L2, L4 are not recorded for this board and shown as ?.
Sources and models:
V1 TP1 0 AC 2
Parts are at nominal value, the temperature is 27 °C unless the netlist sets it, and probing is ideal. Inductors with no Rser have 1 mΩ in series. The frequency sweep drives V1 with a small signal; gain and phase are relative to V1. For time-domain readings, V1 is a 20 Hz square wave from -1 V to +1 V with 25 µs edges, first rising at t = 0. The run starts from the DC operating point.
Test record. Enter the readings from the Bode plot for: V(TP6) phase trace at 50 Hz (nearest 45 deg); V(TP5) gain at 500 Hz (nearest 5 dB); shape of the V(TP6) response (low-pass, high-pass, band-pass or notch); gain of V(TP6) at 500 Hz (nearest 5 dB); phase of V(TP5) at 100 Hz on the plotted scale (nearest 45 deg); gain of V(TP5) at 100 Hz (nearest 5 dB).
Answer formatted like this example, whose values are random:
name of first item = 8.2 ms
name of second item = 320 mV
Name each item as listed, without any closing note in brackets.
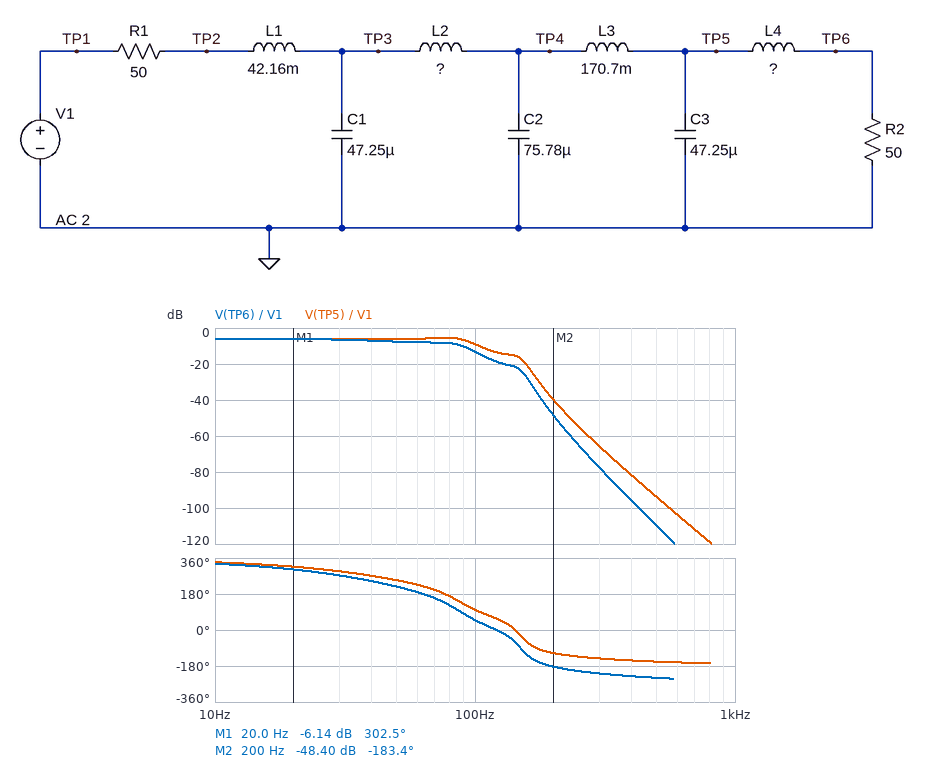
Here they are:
V(TP6) phase trace at 50 Hz = 225 deg
V(TP5) gain at 500 Hz = -95 dB
shape of the V(TP6) response = low-pass
gain of V(TP6) at 500 Hz = -110 dB
phase of V(TP5) at 100 Hz on the plotted scale = 90 deg
gain of V(TP5) at 100 Hz = -10 dB
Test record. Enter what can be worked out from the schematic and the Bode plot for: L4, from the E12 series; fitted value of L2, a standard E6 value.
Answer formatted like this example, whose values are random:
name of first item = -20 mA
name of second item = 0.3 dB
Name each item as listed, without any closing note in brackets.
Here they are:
L4, from the E12 series = 100 mH
fitted value of L2, a standard E6 value = 47 mH
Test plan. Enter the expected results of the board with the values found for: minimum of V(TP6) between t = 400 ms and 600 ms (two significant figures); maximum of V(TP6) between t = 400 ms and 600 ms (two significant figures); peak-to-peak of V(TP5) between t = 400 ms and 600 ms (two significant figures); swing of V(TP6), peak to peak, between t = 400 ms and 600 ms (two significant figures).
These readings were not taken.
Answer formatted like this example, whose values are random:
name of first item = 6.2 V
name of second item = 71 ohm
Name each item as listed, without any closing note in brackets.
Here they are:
minimum of V(TP6) between t = 400 ms and 600 ms = -540 mV
maximum of V(TP6) between t = 400 ms and 600 ms = 540 mV
peak-to-peak of V(TP5) between t = 400 ms and 600 ms = 1.3 V
swing of V(TP6), peak to peak, between t = 400 ms and 600 ms = 1.1 V
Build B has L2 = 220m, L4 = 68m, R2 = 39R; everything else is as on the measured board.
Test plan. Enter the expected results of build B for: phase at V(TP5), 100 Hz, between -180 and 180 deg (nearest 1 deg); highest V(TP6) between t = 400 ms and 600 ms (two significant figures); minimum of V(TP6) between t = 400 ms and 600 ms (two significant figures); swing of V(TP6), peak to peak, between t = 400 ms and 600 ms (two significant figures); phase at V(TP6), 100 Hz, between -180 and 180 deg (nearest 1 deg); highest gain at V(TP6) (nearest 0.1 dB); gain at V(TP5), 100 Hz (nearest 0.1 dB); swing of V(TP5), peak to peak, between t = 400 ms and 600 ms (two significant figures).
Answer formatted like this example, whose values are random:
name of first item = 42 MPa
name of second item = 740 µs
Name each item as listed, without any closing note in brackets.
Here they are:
phase at V(TP5), 100 Hz, between -180 and 180 deg = 2 deg
highest V(TP6) between t = 400 ms and 600 ms = 560 mV
minimum of V(TP6) between t = 400 ms and 600 ms = -560 mV
swing of V(TP6), peak to peak, between t = 400 ms and 600 ms = 1.1 V
phase at V(TP6), 100 Hz, between -180 and 180 deg = -46 deg
highest gain at V(TP6) = -7.1 dB
gain at V(TP5), 100 Hz = -16.4 dB
swing of V(TP5), peak to peak, between t = 400 ms and 600 ms = 1.2 V
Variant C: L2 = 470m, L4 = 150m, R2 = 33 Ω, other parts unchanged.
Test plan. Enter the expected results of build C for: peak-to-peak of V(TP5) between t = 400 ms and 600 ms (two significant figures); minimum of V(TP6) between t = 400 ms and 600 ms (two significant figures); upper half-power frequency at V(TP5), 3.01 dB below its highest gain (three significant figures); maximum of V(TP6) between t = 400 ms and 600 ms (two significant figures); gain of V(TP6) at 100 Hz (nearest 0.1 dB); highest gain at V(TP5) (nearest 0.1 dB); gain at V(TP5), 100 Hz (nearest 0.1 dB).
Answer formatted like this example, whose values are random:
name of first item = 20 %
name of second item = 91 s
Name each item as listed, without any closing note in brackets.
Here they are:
peak-to-peak of V(TP5) between t = 400 ms and 600 ms = 1.1 V
minimum of V(TP6) between t = 400 ms and 600 ms = -410 mV
upper half-power frequency at V(TP5), 3.01 dB below its highest gain = 49.1 Hz
maximum of V(TP6) between t = 400 ms and 600 ms = 410 mV
gain of V(TP6) at 100 Hz = -32.1 dB
highest gain at V(TP5) = -5.1 dB
gain at V(TP5), 100 Hz = -22.5 dB
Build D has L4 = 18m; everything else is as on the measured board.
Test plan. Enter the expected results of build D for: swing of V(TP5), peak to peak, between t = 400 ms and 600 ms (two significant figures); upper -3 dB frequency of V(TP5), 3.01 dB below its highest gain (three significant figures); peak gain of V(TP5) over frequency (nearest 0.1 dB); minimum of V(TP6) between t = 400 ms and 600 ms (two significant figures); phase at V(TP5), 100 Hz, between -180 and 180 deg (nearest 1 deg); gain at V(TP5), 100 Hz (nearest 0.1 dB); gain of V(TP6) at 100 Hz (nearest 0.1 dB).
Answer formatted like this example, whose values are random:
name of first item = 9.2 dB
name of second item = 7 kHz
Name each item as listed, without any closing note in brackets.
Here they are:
swing of V(TP5), peak to peak, between t = 400 ms and 600 ms = 1.1 V
upper -3 dB frequency of V(TP5), 3.01 dB below its highest gain = 70.9 Hz
peak gain of V(TP5) over frequency = -6.0 dB
minimum of V(TP6) between t = 400 ms and 600 ms = -560 mV
phase at V(TP5), 100 Hz, between -180 and 180 deg = 112 deg
gain at V(TP5), 100 Hz = -14.7 dB
gain of V(TP6) at 100 Hz = -14.9 dB
